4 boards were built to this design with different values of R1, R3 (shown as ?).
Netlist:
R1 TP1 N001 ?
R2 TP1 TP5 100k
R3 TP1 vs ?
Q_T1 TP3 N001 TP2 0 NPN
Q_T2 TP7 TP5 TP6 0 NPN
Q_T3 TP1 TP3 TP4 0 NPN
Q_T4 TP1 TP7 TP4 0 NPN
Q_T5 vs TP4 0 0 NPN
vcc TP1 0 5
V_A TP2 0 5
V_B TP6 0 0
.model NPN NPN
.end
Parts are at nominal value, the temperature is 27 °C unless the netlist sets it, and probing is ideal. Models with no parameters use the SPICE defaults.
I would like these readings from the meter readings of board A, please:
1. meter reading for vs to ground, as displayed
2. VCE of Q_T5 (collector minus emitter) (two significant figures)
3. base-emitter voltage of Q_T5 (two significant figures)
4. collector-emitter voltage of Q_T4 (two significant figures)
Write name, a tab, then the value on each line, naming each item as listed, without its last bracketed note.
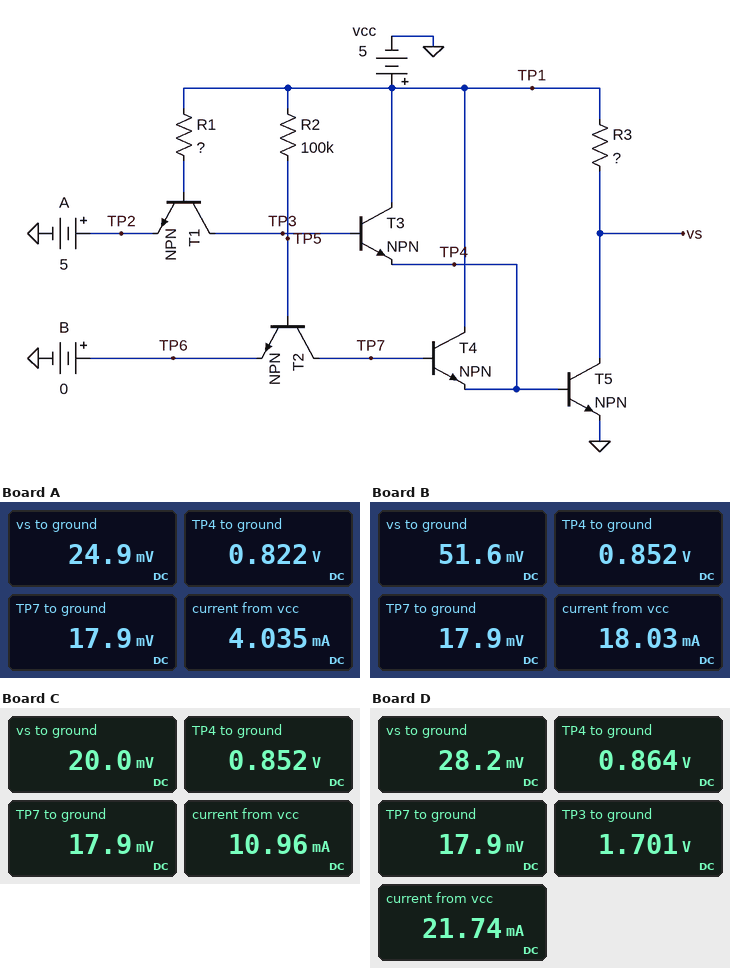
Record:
meter reading for vs to ground, as displayed	24.9 mV
VCE of Q_T5 (collector minus emitter)	25 mV
base-emitter voltage of Q_T5	820 mV
collector-emitter voltage of Q_T4	4.2 V
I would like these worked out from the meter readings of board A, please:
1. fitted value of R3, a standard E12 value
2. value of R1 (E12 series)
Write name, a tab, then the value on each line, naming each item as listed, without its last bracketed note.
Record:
fitted value of R3, a standard E12 value	3.3 kΩ
value of R1	220 kΩ
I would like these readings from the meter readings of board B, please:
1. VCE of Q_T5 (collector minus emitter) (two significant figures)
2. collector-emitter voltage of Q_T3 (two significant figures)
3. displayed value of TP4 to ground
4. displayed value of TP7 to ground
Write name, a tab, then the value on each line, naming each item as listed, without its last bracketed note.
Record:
VCE of Q_T5 (collector minus emitter)	52 mV
collector-emitter voltage of Q_T3	4.1 V
displayed value of TP4 to ground	0.852 V
displayed value of TP7 to ground	17.9 mV
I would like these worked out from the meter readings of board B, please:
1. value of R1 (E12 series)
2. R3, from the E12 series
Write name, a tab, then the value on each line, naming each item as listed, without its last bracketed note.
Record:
value of R1	180 kΩ
R3, from the E12 series	330 Ω
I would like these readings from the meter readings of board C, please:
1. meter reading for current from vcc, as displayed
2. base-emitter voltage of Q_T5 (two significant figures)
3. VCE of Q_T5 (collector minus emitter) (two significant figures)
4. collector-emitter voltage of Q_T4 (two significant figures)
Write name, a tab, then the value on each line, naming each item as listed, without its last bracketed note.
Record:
meter reading for current from vcc, as displayed	10.96 mA
base-emitter voltage of Q_T5	850 mV
VCE of Q_T5 (collector minus emitter)	20 mV
collector-emitter voltage of Q_T4	4.1 V
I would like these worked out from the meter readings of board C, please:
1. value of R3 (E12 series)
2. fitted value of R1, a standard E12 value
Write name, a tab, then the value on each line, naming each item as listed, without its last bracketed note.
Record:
value of R3	3.3 kΩ
fitted value of R1, a standard E12 value	56 kΩ
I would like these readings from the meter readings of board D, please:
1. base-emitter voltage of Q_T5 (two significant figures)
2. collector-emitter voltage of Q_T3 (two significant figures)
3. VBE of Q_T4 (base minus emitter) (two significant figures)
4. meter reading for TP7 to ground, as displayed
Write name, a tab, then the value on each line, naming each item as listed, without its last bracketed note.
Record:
base-emitter voltage of Q_T5	860 mV
collector-emitter voltage of Q_T3	4.1 V
VBE of Q_T4 (base minus emitter)	-850 mV
meter reading for TP7 to ground, as displayed	17.9 mV
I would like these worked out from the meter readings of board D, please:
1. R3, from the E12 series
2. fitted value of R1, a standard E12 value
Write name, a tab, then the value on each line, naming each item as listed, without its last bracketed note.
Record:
R3, from the E12 series	470 Ω
fitted value of R1, a standard E12 value	47 kΩ
